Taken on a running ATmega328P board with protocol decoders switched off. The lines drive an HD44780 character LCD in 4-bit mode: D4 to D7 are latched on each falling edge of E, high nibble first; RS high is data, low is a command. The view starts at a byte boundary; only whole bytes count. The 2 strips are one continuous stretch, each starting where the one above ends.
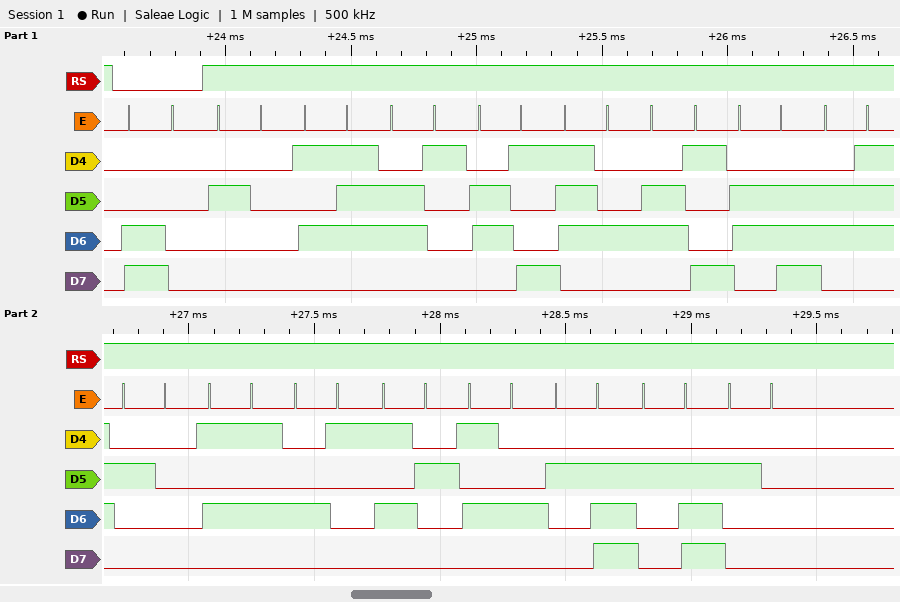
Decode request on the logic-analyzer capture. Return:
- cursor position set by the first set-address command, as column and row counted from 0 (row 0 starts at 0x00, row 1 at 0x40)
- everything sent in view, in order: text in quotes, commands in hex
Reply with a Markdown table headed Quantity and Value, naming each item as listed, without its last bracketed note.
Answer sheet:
| Quantity | Value |
|---|---|
| cursor position set by the first set-address command, as column and row counted from 0 | column 0, row 1 |
| everything sent in view, in order: text in quotes, commands in hex | 0xC0 " Waiting UART.. " |
